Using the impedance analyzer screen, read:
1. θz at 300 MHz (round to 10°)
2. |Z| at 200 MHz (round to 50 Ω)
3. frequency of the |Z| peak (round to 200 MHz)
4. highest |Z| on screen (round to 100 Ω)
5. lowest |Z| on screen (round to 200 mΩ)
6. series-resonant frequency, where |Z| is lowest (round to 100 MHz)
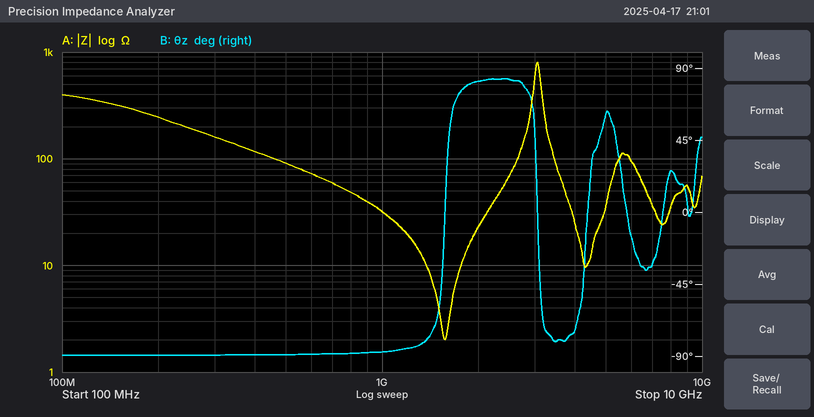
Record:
-90°
250 Ω
3.0 GHz
800 Ω
2.0 Ω
1.6 GHz
